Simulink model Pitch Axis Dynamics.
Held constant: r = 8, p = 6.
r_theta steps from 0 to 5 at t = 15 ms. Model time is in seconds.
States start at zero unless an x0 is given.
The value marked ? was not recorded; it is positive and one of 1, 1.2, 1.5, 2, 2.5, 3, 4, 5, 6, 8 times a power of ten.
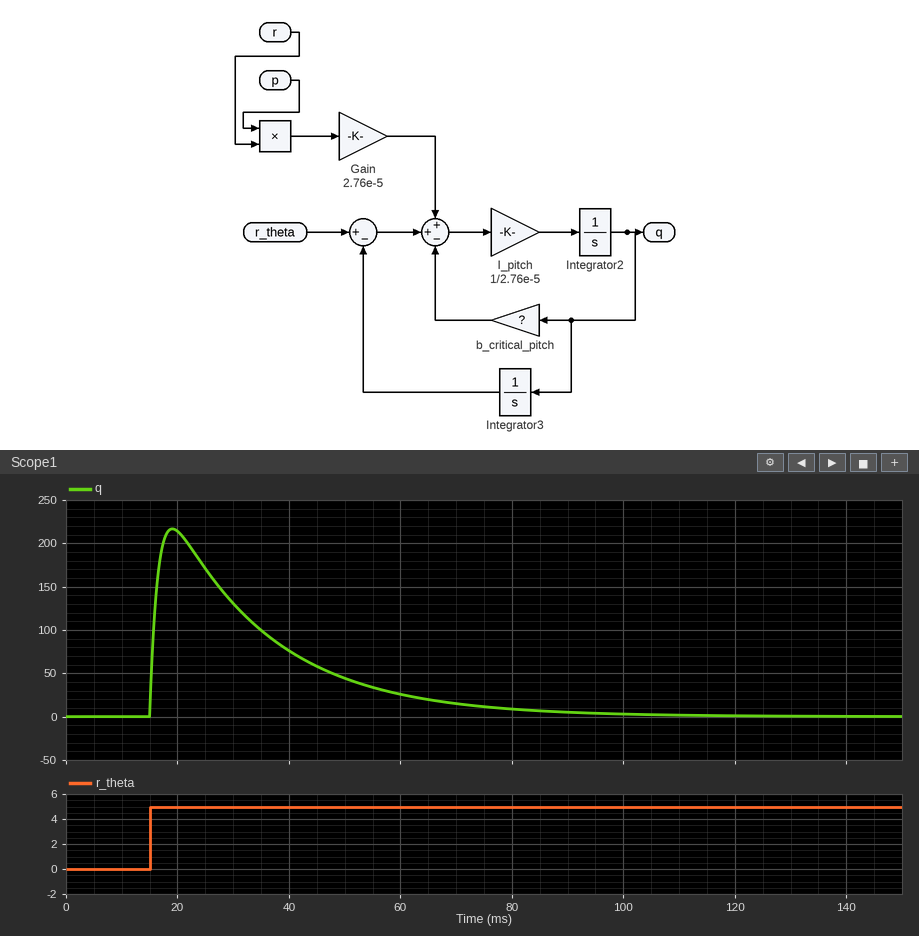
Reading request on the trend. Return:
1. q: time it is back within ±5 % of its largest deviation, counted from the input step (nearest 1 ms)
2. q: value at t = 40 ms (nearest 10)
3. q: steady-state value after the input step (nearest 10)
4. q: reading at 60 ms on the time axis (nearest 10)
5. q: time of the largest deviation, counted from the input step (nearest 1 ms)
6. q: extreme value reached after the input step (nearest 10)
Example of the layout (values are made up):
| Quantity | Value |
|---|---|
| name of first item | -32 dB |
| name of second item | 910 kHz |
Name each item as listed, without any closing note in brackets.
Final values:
| Quantity | Value |
|---|---|
| q: time it is back within ±5 % of its largest deviation, counted from the input step | 61 ms |
| q: value at t = 40 ms | 80 |
| q: steady-state value after the input step | 0 |
| q: reading at 60 ms on the time axis | 30 |
| q: time of the largest deviation, counted from the input step | 4 ms |
| q: extreme value reached after the input step | 220 |
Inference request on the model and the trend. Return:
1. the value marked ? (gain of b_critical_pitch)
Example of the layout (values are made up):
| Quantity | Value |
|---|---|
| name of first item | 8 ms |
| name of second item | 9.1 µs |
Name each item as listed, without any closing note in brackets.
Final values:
| Quantity | Value |
|---|---|
| the value marked ? | 0.02 |
